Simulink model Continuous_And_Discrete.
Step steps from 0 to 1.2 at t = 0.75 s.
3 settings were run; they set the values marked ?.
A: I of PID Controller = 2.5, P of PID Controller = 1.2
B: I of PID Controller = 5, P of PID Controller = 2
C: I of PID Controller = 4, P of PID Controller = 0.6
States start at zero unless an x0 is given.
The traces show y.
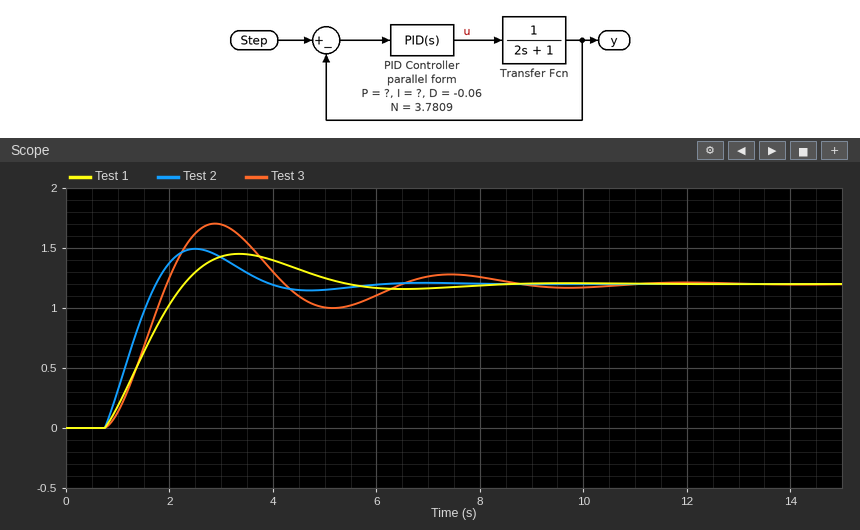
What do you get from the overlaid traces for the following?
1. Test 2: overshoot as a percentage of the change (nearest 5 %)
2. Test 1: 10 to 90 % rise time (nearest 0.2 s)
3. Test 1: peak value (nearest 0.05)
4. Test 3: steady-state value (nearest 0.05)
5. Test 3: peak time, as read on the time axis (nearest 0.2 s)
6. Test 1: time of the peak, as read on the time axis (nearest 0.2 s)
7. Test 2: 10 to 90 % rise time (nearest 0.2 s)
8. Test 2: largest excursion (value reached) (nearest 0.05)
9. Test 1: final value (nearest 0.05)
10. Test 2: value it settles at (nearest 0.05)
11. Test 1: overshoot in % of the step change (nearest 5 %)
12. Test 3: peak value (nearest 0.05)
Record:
25 %
1.2 s
1.45
1.20
2.8 s
3.4 s
0.8 s
1.50
1.20
1.20
20 %
1.70
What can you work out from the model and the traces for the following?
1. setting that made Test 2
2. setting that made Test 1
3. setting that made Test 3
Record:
B
A
C
